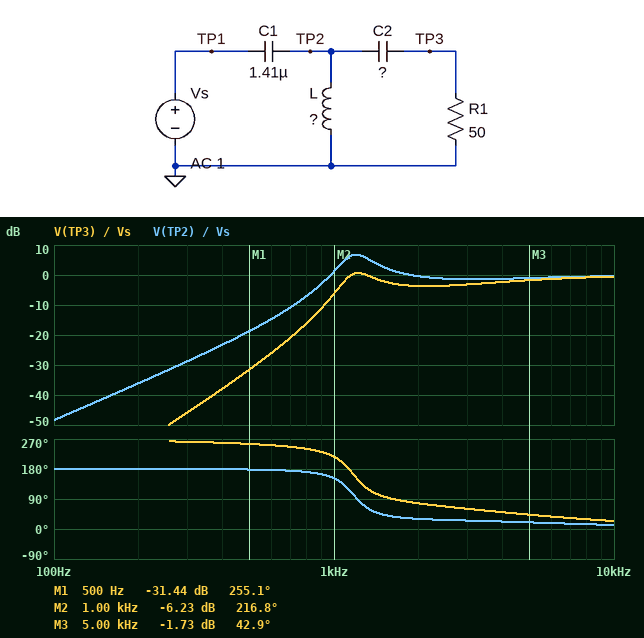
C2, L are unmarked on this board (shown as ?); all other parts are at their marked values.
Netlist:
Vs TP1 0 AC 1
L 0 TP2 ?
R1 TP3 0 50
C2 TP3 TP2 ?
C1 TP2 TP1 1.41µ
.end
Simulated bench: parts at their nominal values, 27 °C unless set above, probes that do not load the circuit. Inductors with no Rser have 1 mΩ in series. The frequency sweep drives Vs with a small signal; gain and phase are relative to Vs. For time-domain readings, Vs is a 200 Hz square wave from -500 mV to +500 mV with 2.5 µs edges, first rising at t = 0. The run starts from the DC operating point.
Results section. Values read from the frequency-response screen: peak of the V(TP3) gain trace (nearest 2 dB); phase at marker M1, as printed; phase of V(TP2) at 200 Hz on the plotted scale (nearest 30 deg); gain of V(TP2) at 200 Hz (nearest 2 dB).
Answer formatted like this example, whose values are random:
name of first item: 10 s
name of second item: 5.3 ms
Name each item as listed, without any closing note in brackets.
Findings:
peak of the V(TP3) gain trace: 0 dB
phase at marker M1, as printed: 255.1 deg
phase of V(TP2) at 200 Hz on the plotted scale: 180 deg
gain of V(TP2) at 200 Hz: -36 dB
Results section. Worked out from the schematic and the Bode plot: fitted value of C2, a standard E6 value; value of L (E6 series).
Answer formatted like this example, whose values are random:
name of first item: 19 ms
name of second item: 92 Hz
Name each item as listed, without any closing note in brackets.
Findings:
fitted value of C2, a standard E6 value: 1.5 µF
value of L: 6.8 mH
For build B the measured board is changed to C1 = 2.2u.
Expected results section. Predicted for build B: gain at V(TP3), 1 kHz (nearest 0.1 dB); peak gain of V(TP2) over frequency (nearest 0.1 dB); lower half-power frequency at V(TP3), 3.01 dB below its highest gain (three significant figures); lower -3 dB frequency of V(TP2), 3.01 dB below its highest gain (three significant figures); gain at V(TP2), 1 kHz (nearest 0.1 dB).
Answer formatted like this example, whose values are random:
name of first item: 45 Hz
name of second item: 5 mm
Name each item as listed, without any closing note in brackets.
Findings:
gain at V(TP3), 1 kHz: 3.2 dB
peak gain of V(TP2) over frequency: 11.4 dB
lower half-power frequency at V(TP3), 3.01 dB below its highest gain: 966 Hz
lower -3 dB frequency of V(TP2), 3.01 dB below its highest gain: 957 Hz
gain at V(TP2), 1 kHz: 10.6 dB
